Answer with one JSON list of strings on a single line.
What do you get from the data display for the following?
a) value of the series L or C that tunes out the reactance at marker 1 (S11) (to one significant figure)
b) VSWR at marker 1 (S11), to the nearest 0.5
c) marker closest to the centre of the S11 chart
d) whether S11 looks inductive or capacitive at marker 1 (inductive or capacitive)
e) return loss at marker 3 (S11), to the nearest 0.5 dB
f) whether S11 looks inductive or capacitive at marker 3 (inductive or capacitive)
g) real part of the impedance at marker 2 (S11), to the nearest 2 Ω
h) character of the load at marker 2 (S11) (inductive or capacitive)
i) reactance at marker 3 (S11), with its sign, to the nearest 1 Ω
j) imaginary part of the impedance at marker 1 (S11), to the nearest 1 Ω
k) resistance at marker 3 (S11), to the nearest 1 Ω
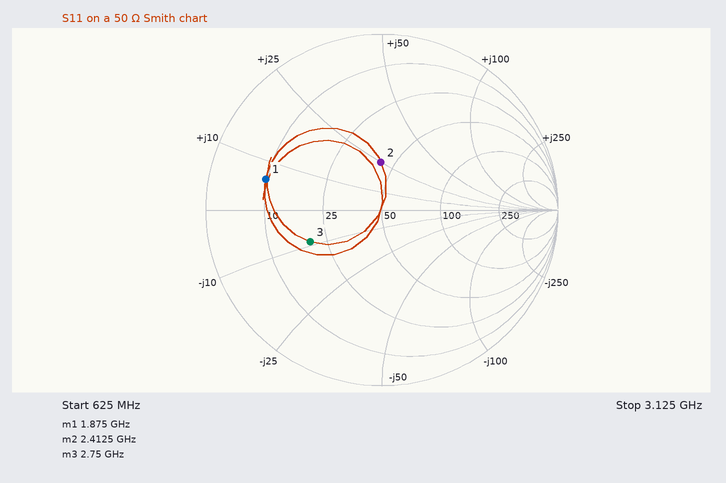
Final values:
["10 pF", "5.5", "marker 2", "inductive", "7.0 dB", "capacitive", "42 Ω", "inductive", "-9 Ω", "+6 Ω", "20 Ω"]
